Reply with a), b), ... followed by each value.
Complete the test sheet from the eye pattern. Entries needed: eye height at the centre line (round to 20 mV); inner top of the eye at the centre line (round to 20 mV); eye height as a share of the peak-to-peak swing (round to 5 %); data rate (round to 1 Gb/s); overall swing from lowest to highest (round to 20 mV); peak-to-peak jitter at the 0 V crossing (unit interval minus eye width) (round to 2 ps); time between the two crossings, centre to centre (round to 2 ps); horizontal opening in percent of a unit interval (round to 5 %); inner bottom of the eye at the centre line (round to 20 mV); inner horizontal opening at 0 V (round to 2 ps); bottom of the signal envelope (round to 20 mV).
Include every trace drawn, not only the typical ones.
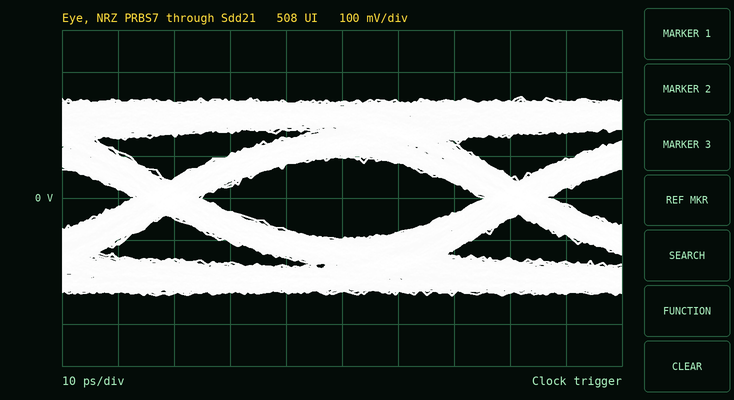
a) 200 mV
b) 100 mV
c) 40 %
d) 16 Gb/s
e) 480 mV
f) 12 ps
g) 62 ps
h) 80 %
i) -100 mV
j) 50 ps
k) -240 mV
